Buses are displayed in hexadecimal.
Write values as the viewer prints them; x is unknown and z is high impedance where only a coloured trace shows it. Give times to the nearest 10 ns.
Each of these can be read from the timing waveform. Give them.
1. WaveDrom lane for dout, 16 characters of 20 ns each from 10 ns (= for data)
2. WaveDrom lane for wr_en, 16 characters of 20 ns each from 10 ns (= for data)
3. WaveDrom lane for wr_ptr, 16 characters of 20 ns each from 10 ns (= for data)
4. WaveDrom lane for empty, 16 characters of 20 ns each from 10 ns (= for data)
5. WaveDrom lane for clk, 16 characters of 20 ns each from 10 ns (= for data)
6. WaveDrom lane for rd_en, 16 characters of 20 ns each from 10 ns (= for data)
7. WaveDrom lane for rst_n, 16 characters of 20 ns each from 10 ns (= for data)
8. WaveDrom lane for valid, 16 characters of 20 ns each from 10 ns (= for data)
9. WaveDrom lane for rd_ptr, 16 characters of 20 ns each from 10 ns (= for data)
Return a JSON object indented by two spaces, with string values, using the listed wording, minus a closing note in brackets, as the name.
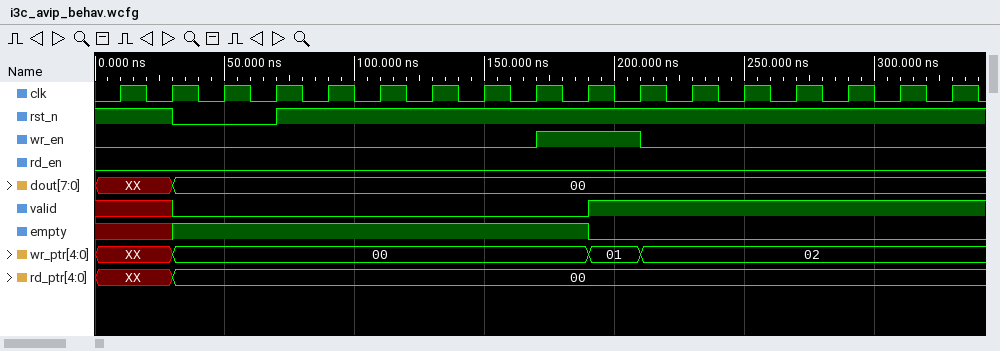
{
  "WaveDrom lane for dout, 16 characters of 20 ns each from 10 ns": "{name: 'dout', wave: 'x=..............', data: '00'}",
  "WaveDrom lane for wr_en, 16 characters of 20 ns each from 10 ns": "{name: 'wr_en', wave: '0.......1.0.....'}",
  "WaveDrom lane for wr_ptr, 16 characters of 20 ns each from 10 ns": "{name: 'wr_ptr', wave: 'x=.......==.....', data: '00 01 02'}",
  "WaveDrom lane for empty, 16 characters of 20 ns each from 10 ns": "{name: 'empty', wave: 'x1.......0......'}",
  "WaveDrom lane for clk, 16 characters of 20 ns each from 10 ns": "{name: 'clk', wave: 'p...............'}",
  "WaveDrom lane for rd_en, 16 characters of 20 ns each from 10 ns": "{name: 'rd_en', wave: '0...............'}",
  "WaveDrom lane for rst_n, 16 characters of 20 ns each from 10 ns": "{name: 'rst_n', wave: '10.1............'}",
  "WaveDrom lane for valid, 16 characters of 20 ns each from 10 ns": "{name: 'valid', wave: 'x0.......1......'}",
  "WaveDrom lane for rd_ptr, 16 characters of 20 ns each from 10 ns": "{name: 'rd_ptr', wave: 'x=..............', data: '00'}"
}
